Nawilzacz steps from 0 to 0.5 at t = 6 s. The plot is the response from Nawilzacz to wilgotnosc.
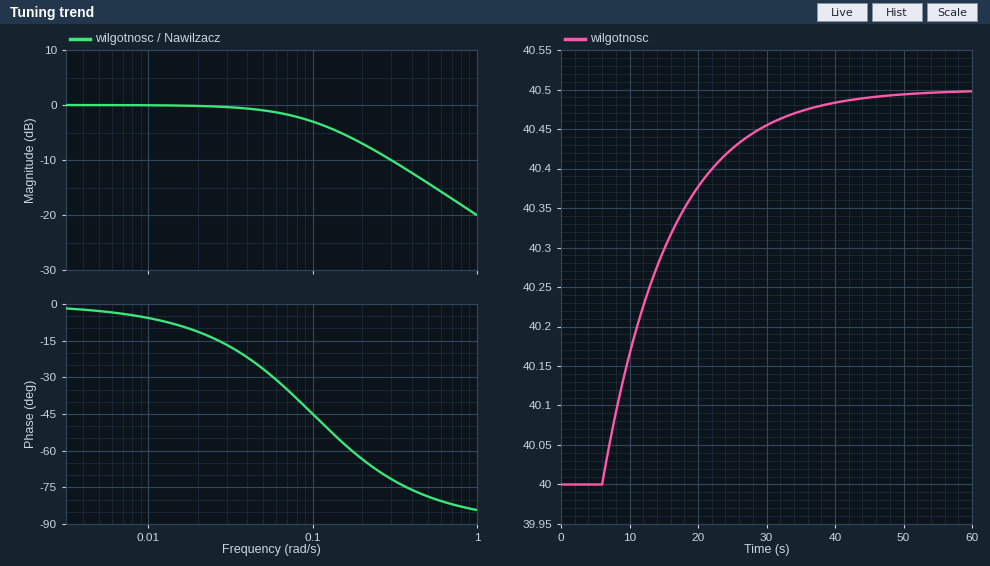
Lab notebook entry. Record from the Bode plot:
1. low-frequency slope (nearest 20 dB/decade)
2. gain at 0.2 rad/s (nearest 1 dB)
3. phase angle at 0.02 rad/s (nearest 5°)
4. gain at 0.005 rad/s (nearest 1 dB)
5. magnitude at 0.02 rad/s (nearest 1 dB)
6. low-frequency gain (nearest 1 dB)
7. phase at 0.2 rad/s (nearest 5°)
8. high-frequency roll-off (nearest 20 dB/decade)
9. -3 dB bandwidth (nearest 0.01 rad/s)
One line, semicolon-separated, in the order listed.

0 dB/decade; -7 dB; -10°; 0 dB; 0 dB; 0 dB; -65°; -20 dB/decade; 0.10 rad/s
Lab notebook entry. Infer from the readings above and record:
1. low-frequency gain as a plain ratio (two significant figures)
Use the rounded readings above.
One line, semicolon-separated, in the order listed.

1.0
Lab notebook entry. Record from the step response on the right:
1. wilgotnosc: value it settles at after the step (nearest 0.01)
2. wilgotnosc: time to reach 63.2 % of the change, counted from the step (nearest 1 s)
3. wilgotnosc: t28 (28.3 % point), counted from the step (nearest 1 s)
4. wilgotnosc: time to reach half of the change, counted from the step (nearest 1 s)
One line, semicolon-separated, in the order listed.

40.50; 10 s; 3 s; 7 s
